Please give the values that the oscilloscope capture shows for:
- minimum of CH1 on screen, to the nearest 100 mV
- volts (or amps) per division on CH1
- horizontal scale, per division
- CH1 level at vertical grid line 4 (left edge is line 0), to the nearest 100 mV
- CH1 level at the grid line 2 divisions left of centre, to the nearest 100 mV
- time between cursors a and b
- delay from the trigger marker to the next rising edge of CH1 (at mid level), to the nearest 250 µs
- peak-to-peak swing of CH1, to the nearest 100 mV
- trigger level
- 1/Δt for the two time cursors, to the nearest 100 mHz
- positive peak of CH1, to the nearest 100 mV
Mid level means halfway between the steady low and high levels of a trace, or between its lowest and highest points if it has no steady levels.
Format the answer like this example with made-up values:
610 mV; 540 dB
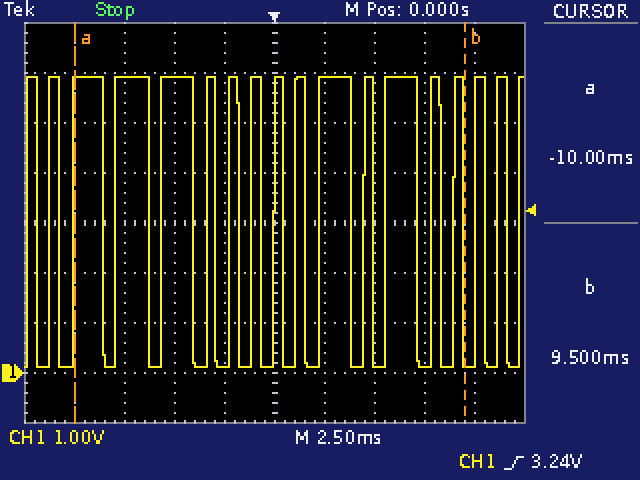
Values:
100 mV; 1 V; 2.5 ms; 100 mV; 5.9 V; 19.50 ms; 1.00 ms; 5.8 V; 3.24 V; 51.3 Hz; 5.9 V
